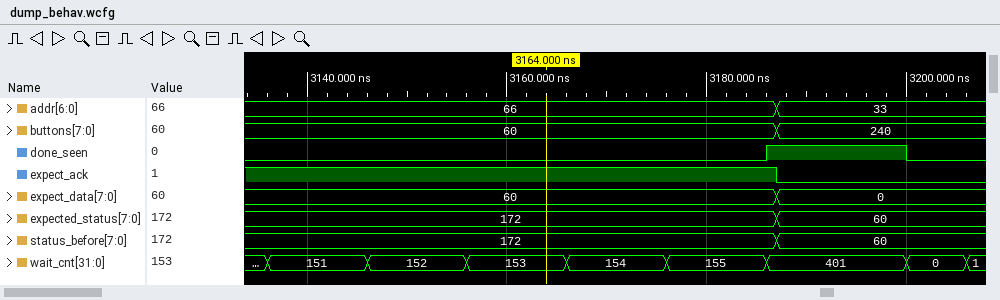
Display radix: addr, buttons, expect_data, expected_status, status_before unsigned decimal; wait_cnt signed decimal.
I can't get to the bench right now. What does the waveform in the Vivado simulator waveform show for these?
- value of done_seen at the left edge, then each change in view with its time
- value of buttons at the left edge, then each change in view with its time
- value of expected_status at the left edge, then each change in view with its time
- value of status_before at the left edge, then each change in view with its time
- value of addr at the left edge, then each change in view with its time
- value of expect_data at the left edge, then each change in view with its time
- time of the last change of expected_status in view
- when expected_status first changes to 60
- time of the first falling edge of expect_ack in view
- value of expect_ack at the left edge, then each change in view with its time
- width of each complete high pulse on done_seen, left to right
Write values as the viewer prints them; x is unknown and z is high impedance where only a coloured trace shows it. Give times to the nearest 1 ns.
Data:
0, 1 at 3186 ns, 0 at 3200 ns
60, 240 at 3187 ns
172, 60 at 3187 ns
172, 60 at 3187 ns
66, 33 at 3187 ns
60, 0 at 3187 ns
3187 ns
3187 ns
3187 ns
1, 0 at 3187 ns
14 ns
